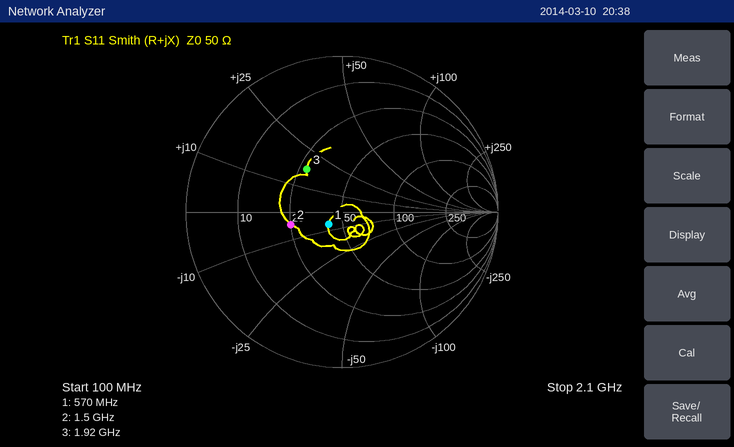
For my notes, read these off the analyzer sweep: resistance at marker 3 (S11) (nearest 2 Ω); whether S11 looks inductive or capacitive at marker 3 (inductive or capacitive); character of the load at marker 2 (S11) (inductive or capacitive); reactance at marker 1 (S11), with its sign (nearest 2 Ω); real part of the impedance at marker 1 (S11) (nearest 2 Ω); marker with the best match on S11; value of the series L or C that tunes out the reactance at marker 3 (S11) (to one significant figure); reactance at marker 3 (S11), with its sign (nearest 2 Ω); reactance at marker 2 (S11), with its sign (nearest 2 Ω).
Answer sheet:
28 Ω
inductive
capacitive
-6 Ω
42 Ω
marker 1
5 pF
+18 Ω
-4 Ω
